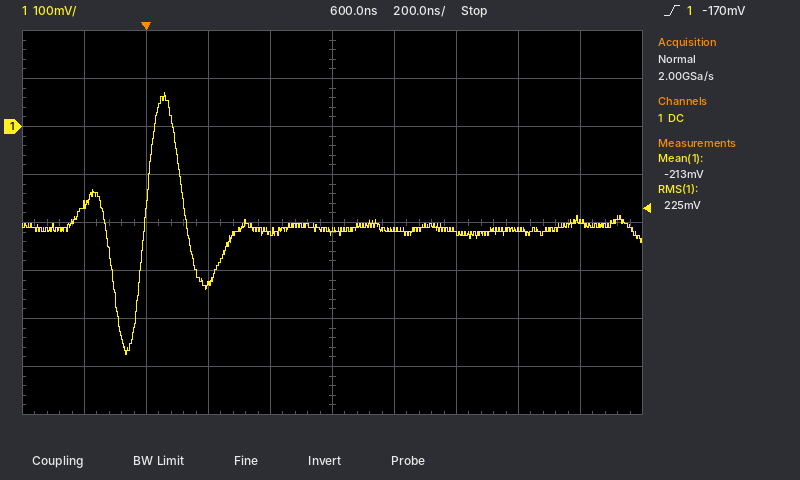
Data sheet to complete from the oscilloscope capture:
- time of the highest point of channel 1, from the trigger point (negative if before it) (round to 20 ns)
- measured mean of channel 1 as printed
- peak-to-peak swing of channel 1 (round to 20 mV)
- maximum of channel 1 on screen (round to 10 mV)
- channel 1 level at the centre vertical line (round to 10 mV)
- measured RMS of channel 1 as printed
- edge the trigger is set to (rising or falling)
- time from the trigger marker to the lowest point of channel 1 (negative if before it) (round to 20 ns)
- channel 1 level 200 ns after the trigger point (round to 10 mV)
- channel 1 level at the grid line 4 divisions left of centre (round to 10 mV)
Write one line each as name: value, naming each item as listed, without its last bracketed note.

time of the highest point of channel 1, from the trigger point (negative if before it): +60 ns
measured mean of channel 1 as printed: -213 mV
peak-to-peak swing of channel 1: 540 mV
maximum of channel 1 on screen: 70 mV
channel 1 level at the centre vertical line: -220 mV
measured RMS of channel 1 as printed: 225 mV
edge the trigger is set to: rising
time from the trigger marker to the lowest point of channel 1 (negative if before it): -60 ns
channel 1 level 200 ns after the trigger point: -330 mV
channel 1 level at the grid line 4 divisions left of centre: -160 mV
